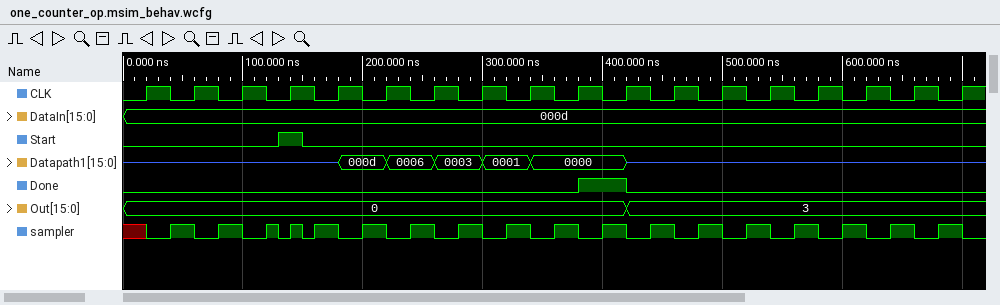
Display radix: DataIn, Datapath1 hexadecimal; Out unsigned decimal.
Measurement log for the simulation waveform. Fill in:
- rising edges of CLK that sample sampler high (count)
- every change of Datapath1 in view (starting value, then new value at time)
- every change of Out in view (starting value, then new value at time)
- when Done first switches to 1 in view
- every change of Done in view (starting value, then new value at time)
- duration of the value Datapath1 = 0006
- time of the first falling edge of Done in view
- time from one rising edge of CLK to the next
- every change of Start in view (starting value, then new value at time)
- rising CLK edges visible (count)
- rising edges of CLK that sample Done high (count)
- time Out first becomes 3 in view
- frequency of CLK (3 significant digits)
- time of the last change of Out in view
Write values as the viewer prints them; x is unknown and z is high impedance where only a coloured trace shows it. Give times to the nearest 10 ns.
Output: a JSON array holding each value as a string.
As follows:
["16", "z, 000d at 180 ns, 0006 at 220 ns, 0003 at 260 ns, 0001 at 300 ns, 0000 at 340 ns, z at 420 ns", "0, 3 at 420 ns", "380 ns", "0, 1 at 380 ns, 0 at 420 ns", "40 ns", "420 ns", "40 ns", "0, 1 at 130 ns, 0 at 150 ns", "18", "1", "420 ns", "25.0 MHz", "420 ns"]
